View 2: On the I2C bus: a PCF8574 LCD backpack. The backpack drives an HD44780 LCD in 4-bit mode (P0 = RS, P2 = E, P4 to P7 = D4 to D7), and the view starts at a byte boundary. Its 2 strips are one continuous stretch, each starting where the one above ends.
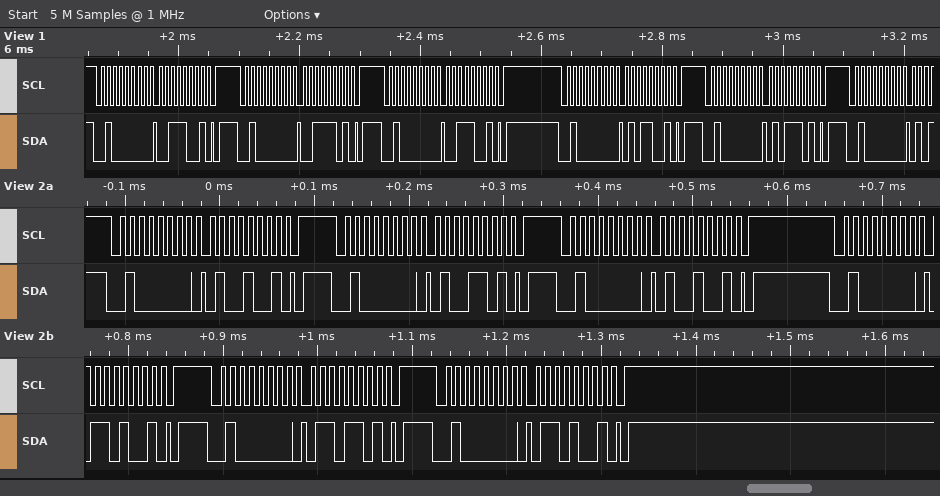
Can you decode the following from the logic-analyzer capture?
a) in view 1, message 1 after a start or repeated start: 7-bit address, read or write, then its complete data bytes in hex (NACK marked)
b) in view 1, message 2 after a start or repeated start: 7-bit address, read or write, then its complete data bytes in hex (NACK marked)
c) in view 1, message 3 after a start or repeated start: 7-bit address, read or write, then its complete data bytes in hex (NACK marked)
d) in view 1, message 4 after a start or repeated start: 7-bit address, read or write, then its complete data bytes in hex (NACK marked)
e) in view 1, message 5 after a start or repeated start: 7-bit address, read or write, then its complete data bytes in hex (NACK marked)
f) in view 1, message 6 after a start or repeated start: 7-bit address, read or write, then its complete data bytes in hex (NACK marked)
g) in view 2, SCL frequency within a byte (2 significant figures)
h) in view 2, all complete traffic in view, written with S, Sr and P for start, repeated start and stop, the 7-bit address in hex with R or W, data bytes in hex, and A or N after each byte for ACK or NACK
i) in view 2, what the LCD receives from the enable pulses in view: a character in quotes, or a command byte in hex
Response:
0x20 write: 39
0x20 write: 3D
0x20 write: 39
0x20 write: 59
0x20 write: 5D
0x20 write
100 kHz
S 20W A 49 A P S 20W A 4D A P S 20W A 49 A P S 20W A 69 A P S 20W A 6D A P S 20W A 69 A P
'F'
